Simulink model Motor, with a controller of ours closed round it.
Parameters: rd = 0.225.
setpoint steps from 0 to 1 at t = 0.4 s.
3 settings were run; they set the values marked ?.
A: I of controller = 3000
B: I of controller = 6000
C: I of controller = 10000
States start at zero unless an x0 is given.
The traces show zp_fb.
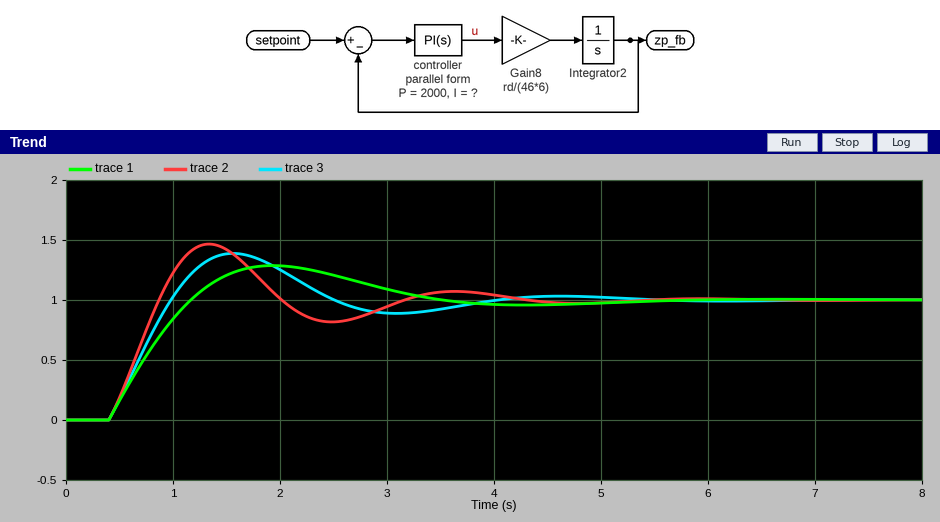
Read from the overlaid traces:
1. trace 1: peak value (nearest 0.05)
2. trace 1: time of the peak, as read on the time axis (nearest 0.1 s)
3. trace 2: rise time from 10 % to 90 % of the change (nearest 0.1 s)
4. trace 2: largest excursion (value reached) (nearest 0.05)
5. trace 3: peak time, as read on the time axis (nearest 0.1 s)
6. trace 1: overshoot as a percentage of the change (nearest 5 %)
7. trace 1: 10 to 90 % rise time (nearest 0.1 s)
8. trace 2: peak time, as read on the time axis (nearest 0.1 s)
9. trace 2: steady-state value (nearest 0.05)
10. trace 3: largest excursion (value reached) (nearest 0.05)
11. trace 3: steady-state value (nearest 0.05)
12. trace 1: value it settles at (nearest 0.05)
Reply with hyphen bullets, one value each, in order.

- 1.30
- 1.9 s
- 0.4 s
- 1.45
- 1.6 s
- 30 %
- 0.6 s
- 1.3 s
- 1.00
- 1.40
- 1.00
- 1.00
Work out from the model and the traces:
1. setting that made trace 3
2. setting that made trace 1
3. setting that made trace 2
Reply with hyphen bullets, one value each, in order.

- B
- A
- C
